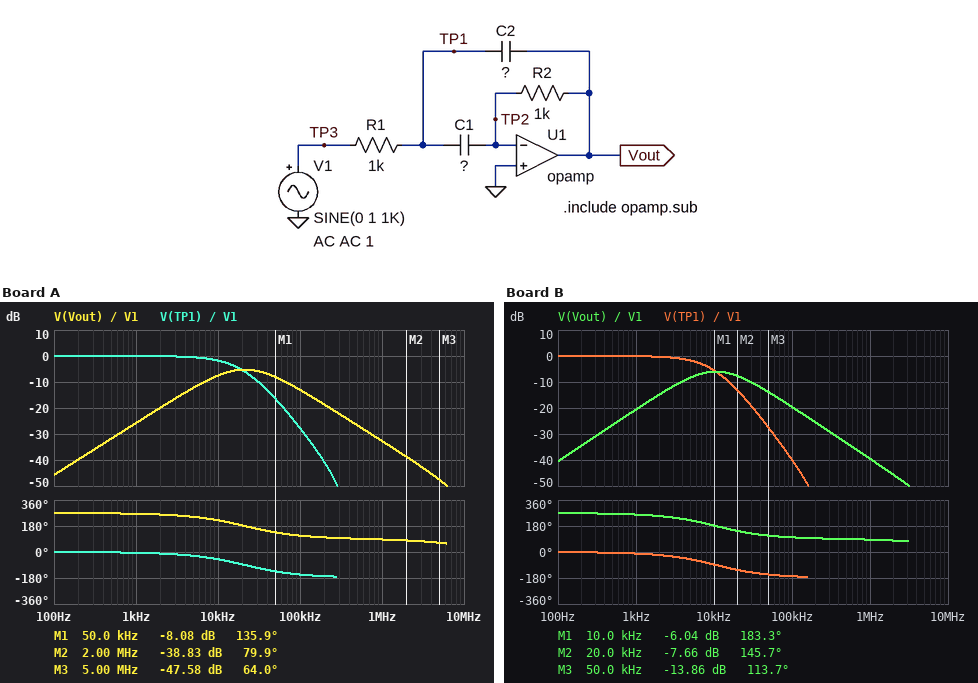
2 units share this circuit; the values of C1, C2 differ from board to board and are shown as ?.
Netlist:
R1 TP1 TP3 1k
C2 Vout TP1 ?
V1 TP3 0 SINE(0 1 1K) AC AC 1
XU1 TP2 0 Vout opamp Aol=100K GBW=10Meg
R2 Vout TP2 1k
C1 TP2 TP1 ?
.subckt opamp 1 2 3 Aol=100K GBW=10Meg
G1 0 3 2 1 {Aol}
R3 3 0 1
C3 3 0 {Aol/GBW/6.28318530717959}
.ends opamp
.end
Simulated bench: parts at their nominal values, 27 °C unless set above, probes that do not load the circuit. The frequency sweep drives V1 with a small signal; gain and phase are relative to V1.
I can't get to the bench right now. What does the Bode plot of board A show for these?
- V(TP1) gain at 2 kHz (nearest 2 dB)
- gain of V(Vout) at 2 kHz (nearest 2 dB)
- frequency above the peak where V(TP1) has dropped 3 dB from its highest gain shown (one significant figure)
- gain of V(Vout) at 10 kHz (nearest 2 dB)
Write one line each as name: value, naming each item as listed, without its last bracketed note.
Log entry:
V(TP1) gain at 2 kHz: 0 dB
gain of V(Vout) at 2 kHz: -20 dB
frequency above the peak where V(TP1) has dropped 3 dB from its highest gain shown: 10 kHz
gain of V(Vout) at 10 kHz: -8 dB
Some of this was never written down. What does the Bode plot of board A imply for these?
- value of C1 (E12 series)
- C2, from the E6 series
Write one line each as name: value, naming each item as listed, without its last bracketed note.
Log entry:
value of C1: 8.2 nF
C2, from the E6 series: 6.8 nF
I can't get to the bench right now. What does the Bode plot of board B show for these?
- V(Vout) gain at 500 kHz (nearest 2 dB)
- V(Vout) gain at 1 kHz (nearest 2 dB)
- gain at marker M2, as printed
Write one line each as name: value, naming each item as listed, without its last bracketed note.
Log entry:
V(Vout) gain at 500 kHz: -34 dB
V(Vout) gain at 1 kHz: -20 dB
gain at marker M2, as printed: -7.66 dB
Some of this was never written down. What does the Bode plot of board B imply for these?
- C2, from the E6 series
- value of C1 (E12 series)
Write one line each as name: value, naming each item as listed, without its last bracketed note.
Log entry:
C2, from the E6 series: 15 nF
value of C1: 15 nF
